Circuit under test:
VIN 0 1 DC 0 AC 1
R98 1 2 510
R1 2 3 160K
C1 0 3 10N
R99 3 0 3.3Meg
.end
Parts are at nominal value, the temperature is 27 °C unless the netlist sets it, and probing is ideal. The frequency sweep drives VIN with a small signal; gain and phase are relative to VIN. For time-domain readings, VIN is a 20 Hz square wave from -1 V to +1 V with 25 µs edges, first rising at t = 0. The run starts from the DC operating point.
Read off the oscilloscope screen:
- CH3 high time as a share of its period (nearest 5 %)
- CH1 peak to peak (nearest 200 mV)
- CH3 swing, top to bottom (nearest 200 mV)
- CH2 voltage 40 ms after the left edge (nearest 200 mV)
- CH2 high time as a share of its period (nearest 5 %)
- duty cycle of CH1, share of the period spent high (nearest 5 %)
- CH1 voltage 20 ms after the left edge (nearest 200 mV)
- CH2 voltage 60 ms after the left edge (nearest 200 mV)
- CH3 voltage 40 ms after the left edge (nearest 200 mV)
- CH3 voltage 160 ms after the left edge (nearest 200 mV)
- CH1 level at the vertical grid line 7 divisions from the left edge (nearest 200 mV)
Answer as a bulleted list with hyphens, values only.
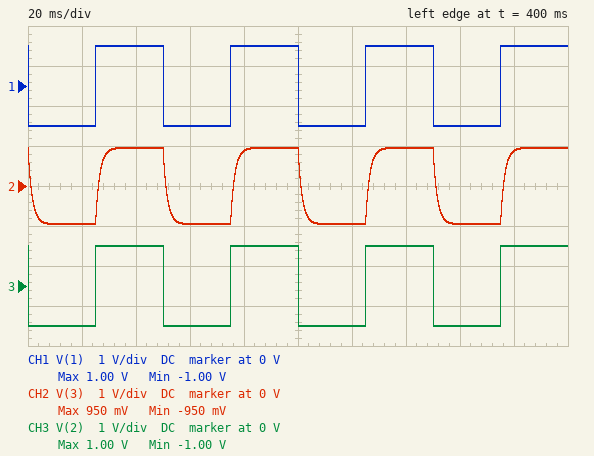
- 50 %
- 2.0 V
- 2.0 V
- 1.0 V
- 50 %
- 50 %
- -1.0 V
- -1.0 V
- 1.0 V
- -1.0 V
- 1.0 V
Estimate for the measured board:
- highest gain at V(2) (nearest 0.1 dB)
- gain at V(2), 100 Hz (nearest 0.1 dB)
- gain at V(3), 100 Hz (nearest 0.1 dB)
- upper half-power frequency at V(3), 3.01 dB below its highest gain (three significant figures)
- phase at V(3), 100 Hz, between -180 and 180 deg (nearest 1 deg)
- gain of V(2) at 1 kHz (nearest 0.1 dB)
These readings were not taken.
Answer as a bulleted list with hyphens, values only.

- 0 dB
- 0 dB
- -3.3 dB
- 104 Hz
- 136 deg
- 0 dB
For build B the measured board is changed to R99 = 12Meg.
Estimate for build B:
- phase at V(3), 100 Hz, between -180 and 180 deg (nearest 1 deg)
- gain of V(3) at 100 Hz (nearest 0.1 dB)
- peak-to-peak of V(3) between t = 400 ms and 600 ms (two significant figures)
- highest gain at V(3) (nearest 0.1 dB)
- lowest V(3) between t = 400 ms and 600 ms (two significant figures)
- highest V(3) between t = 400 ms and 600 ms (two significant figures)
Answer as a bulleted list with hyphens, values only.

- 135 deg
- -3.1 dB
- 2.0 V
- -0.1 dB
- -990 mV
- 990 mV
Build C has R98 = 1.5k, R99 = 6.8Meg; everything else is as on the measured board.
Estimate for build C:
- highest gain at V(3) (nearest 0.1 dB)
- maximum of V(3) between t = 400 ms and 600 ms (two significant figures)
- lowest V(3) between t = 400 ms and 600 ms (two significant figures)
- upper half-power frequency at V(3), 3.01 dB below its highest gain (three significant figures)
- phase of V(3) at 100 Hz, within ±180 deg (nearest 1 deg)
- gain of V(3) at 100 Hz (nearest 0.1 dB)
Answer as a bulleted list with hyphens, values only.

- -0.2 dB
- 980 mV
- -980 mV
- 101 Hz
- 135 deg
- -3.2 dB
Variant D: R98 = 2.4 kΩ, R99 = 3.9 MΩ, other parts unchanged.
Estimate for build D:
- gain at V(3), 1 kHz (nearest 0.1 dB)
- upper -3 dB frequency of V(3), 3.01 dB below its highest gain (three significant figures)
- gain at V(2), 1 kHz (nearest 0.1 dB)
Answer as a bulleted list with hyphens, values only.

- -20.2 dB
- 102 Hz
- -0.1 dB
